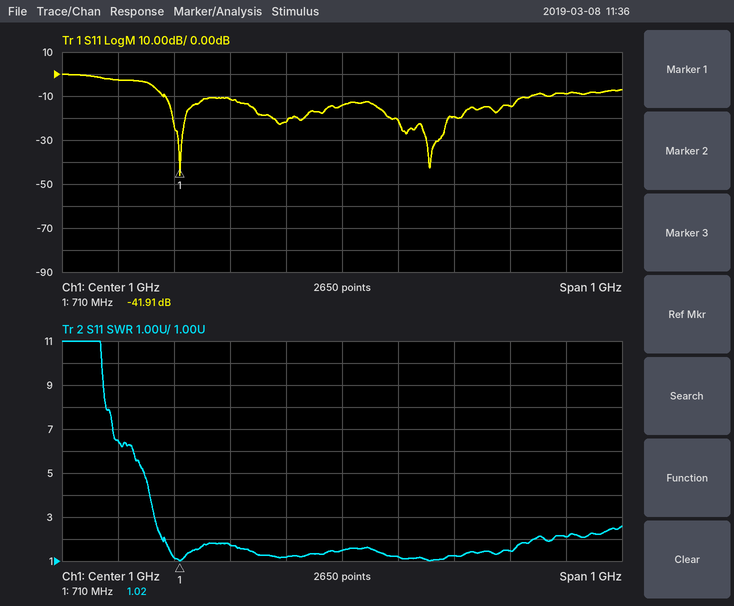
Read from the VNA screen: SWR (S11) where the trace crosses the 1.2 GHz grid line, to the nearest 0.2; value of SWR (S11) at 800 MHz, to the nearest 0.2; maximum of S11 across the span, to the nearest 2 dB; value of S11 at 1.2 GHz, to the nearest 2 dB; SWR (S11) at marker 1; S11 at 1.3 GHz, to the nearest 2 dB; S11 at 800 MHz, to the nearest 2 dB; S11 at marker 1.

1.2
1.8
0 dB
-20 dB
1.02
-14 dB
-12 dB
-41.91 dB
